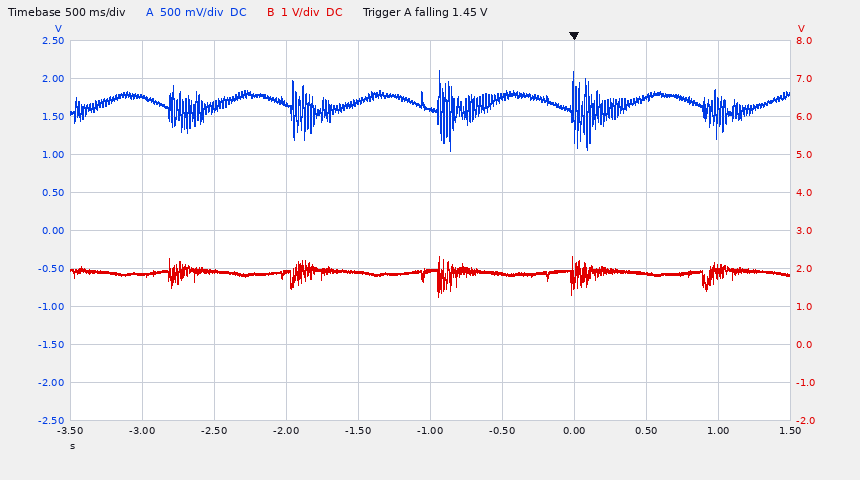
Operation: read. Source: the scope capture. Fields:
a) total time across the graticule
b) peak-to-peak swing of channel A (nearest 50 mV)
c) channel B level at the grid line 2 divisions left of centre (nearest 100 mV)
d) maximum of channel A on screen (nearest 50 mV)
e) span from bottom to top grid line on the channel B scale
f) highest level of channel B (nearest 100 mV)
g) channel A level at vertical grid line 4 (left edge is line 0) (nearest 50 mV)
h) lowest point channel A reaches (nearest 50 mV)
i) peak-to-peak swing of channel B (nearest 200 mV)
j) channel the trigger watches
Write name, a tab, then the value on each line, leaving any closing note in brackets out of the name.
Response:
total time across the graticule	5 s
peak-to-peak swing of channel A	1.05 V
channel B level at the grid line 2 divisions left of centre	1.9 V
maximum of channel A on screen	2.10 V
span from bottom to top grid line on the channel B scale	10 V
highest level of channel B	2.3 V
channel A level at vertical grid line 4 (left edge is line 0)	1.70 V
lowest point channel A reaches	1.05 V
peak-to-peak swing of channel B	1.0 V
channel the trigger watches	channel A
